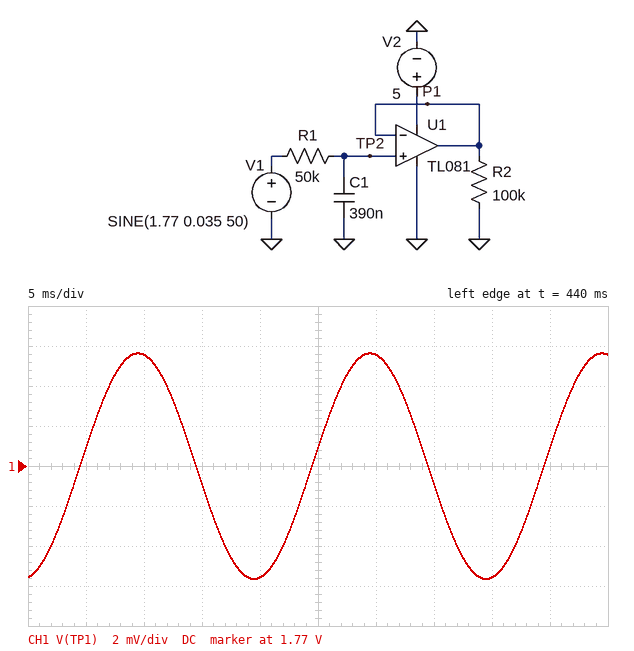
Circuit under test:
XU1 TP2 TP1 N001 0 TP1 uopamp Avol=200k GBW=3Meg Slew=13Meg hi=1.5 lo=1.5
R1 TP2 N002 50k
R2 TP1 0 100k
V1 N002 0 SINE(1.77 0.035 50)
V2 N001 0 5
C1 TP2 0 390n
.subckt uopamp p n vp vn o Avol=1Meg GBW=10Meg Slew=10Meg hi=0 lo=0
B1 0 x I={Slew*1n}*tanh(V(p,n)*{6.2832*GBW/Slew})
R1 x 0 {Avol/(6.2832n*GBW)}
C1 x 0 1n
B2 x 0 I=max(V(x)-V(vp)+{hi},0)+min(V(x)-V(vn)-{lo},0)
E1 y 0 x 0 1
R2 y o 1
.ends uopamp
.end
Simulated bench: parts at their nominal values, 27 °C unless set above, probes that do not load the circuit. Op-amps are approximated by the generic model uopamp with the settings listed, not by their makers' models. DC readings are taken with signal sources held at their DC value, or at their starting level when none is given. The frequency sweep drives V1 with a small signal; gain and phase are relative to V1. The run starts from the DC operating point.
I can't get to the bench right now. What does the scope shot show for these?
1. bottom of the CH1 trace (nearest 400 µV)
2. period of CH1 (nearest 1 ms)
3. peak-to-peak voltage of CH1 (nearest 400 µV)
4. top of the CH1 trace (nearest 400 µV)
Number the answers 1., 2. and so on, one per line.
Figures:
1. 1.7644 V
2. 20 ms
3. 11.2 mV
4. 1.7756 V
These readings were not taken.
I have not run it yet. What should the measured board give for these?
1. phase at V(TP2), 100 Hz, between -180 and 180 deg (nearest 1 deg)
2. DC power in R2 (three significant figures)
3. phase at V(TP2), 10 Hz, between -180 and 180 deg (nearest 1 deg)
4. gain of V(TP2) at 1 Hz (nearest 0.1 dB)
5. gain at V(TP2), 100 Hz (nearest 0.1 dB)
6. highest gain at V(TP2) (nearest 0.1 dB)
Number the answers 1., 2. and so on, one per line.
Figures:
1. -85 deg
2. 31.3 µW
3. -51 deg
4. -0.1 dB
5. -21.8 dB
6. 0 dB
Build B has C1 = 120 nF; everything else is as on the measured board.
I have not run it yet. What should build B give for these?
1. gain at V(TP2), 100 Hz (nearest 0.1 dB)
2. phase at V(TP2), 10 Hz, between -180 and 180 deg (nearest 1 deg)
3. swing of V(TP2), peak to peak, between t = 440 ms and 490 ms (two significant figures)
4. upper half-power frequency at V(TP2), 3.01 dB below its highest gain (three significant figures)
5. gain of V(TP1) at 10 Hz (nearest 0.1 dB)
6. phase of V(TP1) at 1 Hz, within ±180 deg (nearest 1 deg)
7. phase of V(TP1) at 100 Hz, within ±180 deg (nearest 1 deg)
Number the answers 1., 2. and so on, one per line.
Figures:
1. -11.8 dB
2. -21 deg
3. 33 mV
4. 26.5 Hz
5. -0.6 dB
6. -2 deg
7. -75 deg
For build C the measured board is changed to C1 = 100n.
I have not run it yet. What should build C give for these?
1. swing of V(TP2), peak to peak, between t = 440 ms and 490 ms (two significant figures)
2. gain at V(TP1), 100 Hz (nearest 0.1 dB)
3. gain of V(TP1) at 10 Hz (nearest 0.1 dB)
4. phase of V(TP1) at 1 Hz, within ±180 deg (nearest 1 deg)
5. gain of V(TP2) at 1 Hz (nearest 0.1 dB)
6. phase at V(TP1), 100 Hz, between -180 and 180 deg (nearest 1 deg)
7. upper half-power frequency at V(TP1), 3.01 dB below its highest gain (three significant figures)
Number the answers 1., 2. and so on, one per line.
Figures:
1. 38 mV
2. -10.4 dB
3. -0.4 dB
4. -2 deg
5. 0 dB
6. -72 deg
7. 31.8 Hz
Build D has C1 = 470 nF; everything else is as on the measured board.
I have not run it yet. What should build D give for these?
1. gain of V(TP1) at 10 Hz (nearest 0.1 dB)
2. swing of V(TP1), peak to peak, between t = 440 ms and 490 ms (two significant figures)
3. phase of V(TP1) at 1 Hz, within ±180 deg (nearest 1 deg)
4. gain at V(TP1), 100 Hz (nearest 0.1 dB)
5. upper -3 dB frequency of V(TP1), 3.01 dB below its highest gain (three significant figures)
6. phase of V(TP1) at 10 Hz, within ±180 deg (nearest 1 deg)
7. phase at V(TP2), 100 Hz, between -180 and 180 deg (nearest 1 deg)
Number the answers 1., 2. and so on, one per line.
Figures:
1. -5.0 dB
2. 9.4 mV
3. -8 deg
4. -23.4 dB
5. 6.77 Hz
6. -56 deg
7. -86 deg
